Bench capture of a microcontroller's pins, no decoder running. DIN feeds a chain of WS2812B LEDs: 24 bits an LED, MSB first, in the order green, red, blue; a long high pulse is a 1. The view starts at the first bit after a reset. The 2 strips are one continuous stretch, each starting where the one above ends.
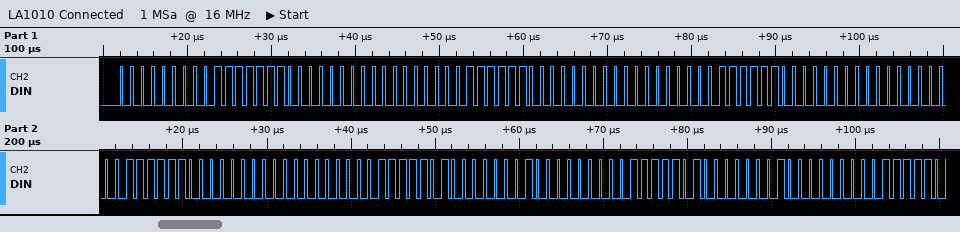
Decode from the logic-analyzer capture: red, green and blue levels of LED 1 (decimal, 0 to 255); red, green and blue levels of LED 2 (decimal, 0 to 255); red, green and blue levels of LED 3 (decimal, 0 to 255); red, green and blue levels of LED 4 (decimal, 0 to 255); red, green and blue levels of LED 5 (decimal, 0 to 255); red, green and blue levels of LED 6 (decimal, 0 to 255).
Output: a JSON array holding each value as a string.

["127, 0, 0", "126, 0, 0", "126, 0, 0", "126, 0, 0", "125, 0, 1", "125, 0, 1"]
